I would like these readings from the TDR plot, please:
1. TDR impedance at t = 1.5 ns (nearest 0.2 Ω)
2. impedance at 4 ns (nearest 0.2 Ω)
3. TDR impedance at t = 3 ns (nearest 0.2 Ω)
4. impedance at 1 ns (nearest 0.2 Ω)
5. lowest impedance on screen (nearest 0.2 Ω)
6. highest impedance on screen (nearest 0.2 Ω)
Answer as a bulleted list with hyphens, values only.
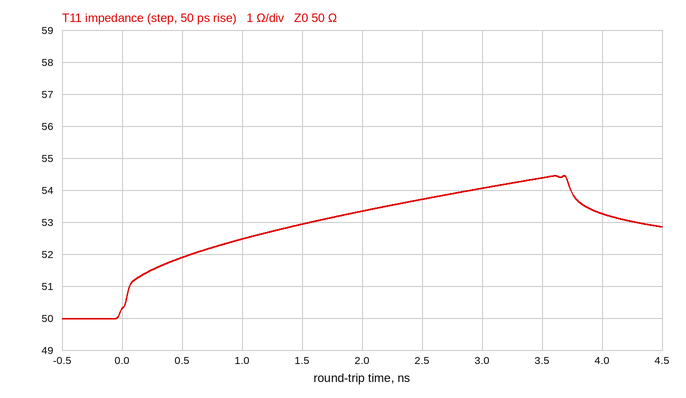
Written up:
- 53.0 Ω
- 53.2 Ω
- 54.0 Ω
- 52.4 Ω
- 50.0 Ω
- 54.4 Ω
